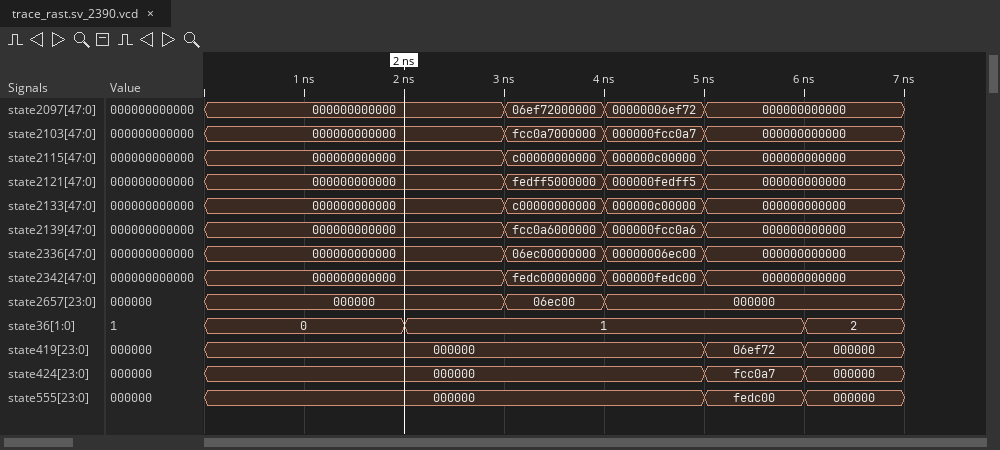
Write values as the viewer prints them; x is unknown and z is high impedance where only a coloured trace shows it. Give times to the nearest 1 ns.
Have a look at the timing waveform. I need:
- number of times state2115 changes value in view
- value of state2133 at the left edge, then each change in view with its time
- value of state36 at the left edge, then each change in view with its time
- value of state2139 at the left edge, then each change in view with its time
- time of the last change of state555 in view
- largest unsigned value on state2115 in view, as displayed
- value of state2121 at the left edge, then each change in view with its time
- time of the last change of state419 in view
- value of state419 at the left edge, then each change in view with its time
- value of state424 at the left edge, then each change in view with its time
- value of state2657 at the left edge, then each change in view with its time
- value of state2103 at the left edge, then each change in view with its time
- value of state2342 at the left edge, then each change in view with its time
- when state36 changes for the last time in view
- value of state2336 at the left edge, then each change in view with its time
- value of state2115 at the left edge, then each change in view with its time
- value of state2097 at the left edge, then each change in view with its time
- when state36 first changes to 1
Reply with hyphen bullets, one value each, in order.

- 3
- 000000000000, c00000000000 at 3 ns, 000000c00000 at 4 ns, 000000000000 at 5 ns
- 0, 1 at 2 ns, 2 at 6 ns
- 000000000000, fcc0a6000000 at 3 ns, 000000fcc0a6 at 4 ns, 000000000000 at 5 ns
- 6 ns
- c00000000000
- 000000000000, fedff5000000 at 3 ns, 000000fedff5 at 4 ns, 000000000000 at 5 ns
- 6 ns
- 000000, 06ef72 at 5 ns, 000000 at 6 ns
- 000000, fcc0a7 at 5 ns, 000000 at 6 ns
- 000000, 06ec00 at 3 ns, 000000 at 4 ns
- 000000000000, fcc0a7000000 at 3 ns, 000000fcc0a7 at 4 ns, 000000000000 at 5 ns
- 000000000000, fedc00000000 at 3 ns, 000000fedc00 at 4 ns, 000000000000 at 5 ns
- 6 ns
- 000000000000, 06ec00000000 at 3 ns, 00000006ec00 at 4 ns, 000000000000 at 5 ns
- 000000000000, c00000000000 at 3 ns, 000000c00000 at 4 ns, 000000000000 at 5 ns
- 000000000000, 06ef72000000 at 3 ns, 00000006ef72 at 4 ns, 000000000000 at 5 ns
- 2 ns
